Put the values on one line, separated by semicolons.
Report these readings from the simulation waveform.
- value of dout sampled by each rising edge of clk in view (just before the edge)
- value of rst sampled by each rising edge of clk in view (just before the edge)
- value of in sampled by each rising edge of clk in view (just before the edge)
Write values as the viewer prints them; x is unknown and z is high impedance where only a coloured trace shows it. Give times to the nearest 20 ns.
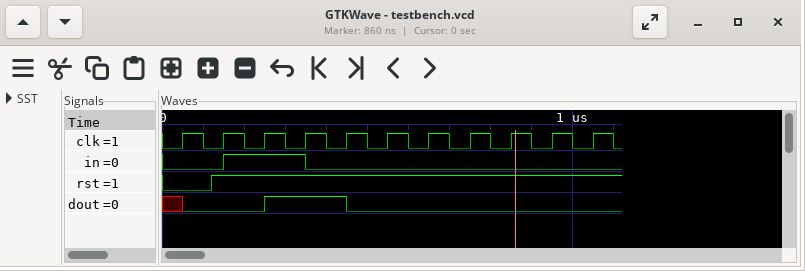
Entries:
x 0 0 1 1 0 0 0 0 0 0; 0 1 1 1 1 1 1 1 1 1 1; 0 0 1 1 0 0 0 0 0 0 0
